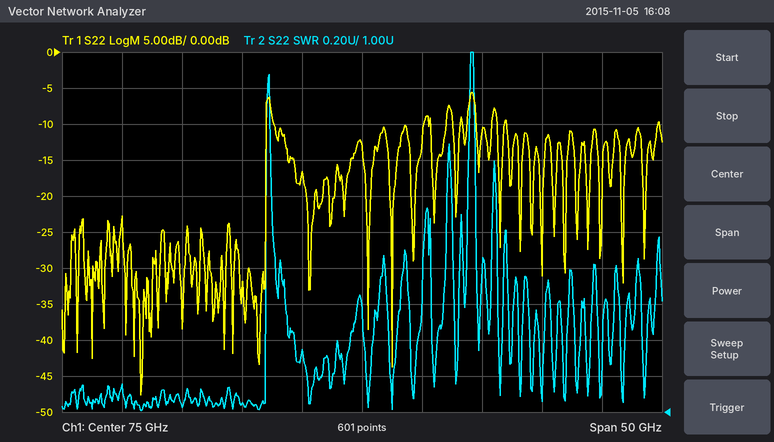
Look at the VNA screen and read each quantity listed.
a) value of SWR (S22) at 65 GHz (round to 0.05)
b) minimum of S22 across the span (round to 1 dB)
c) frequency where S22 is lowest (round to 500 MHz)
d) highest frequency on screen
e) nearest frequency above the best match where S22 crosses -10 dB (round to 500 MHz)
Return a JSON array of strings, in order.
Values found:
["1.05", "-48 dB", "56.5 GHz", "100 GHz", "67.0 GHz"]
